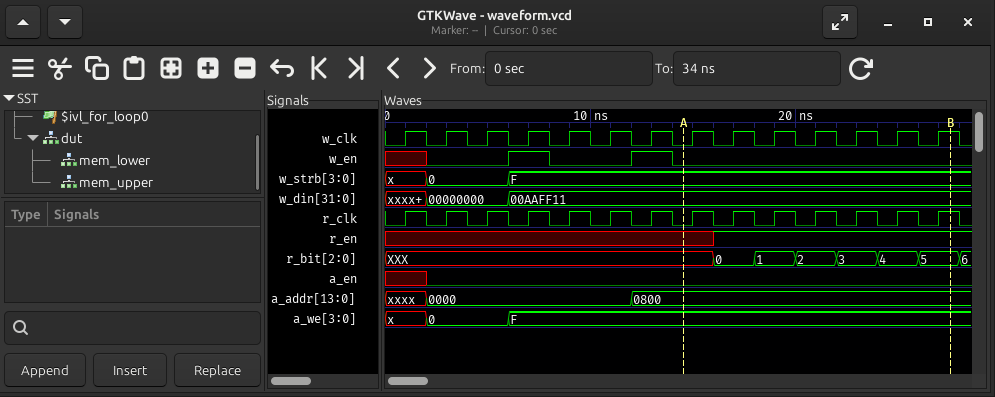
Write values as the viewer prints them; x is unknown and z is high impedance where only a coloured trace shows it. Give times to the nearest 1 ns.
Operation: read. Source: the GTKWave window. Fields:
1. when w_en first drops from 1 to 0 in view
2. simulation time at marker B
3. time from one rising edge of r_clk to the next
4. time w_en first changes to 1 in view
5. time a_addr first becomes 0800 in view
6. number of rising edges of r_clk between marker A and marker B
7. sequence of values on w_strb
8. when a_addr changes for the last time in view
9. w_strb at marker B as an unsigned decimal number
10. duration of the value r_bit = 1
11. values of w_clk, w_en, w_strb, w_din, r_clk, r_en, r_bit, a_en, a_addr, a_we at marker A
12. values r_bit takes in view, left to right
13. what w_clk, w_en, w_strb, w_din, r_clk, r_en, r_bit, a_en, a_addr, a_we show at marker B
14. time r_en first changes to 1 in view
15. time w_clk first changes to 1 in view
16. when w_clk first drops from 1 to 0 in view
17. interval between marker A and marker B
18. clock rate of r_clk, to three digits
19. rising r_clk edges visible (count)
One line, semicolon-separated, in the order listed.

8 ns; 28 ns; 2 ns; 6 ns; 12 ns; 7; x, 0, F; 12 ns; 15; 2 ns; w_clk=0, w_en=0, w_strb=F, w_din=00AAFF11, r_clk=0, r_en=x, r_bit=XXX, a_en=0, a_addr=0800, a_we=F; XXX, 0, 1, 2, 3, 4, 5, 6; w_clk=1, w_en=0, w_strb=F, w_din=00AAFF11, r_clk=1, r_en=1, r_bit=5, a_en=0, a_addr=0800, a_we=F; 16 ns; 1 ns; 2 ns; 13 ns; 500 MHz; 14
